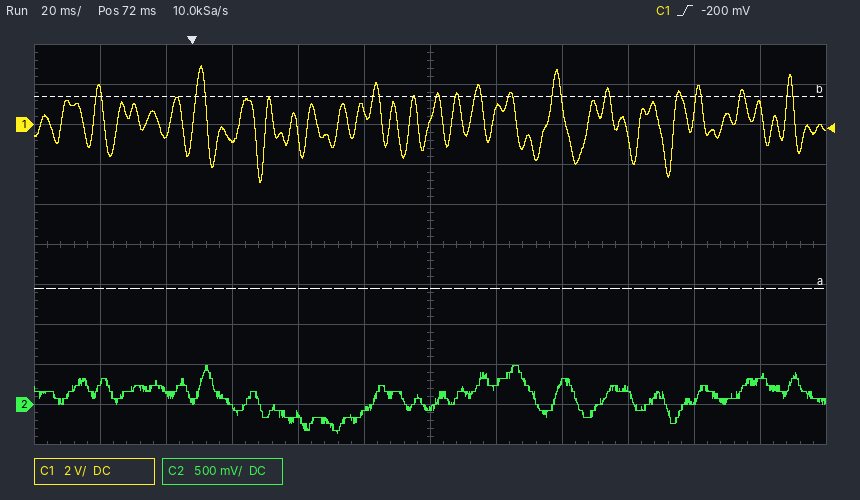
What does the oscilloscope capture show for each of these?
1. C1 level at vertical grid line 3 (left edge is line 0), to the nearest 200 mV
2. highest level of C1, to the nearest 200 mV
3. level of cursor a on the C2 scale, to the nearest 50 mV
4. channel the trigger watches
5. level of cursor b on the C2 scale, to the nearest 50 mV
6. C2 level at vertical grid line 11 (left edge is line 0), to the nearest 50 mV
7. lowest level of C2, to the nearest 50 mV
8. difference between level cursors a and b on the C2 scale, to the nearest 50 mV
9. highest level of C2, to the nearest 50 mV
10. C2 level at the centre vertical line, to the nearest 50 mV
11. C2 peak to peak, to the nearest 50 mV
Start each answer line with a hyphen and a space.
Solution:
- -800 mV
- 3.0 V
- 1.45 V
- C1
- 3.85 V
- 350 mV
- -350 mV
- 2.40 V
- 500 mV
- -50 mV
- 850 mV
